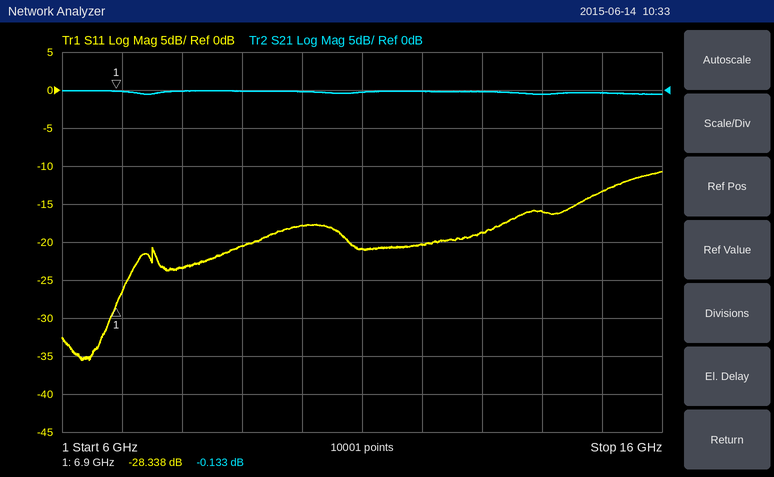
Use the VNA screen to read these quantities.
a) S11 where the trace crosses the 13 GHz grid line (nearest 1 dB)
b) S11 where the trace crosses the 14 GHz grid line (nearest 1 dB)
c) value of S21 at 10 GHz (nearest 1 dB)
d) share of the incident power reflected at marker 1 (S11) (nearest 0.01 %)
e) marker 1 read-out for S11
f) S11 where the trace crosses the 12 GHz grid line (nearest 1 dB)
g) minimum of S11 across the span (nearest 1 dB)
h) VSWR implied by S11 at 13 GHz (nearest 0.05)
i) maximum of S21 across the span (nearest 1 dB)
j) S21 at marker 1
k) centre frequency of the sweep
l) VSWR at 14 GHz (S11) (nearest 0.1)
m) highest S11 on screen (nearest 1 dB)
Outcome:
-19 dB
-16 dB
0 dB
0.15 %
-28.338 dB
-20 dB
-36 dB
1.25
0 dB
-0.133 dB
11 GHz
1.4
-11 dB
